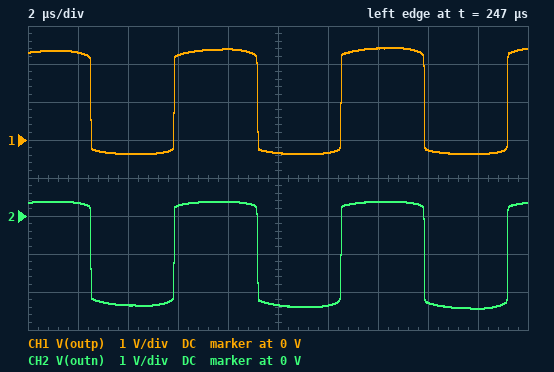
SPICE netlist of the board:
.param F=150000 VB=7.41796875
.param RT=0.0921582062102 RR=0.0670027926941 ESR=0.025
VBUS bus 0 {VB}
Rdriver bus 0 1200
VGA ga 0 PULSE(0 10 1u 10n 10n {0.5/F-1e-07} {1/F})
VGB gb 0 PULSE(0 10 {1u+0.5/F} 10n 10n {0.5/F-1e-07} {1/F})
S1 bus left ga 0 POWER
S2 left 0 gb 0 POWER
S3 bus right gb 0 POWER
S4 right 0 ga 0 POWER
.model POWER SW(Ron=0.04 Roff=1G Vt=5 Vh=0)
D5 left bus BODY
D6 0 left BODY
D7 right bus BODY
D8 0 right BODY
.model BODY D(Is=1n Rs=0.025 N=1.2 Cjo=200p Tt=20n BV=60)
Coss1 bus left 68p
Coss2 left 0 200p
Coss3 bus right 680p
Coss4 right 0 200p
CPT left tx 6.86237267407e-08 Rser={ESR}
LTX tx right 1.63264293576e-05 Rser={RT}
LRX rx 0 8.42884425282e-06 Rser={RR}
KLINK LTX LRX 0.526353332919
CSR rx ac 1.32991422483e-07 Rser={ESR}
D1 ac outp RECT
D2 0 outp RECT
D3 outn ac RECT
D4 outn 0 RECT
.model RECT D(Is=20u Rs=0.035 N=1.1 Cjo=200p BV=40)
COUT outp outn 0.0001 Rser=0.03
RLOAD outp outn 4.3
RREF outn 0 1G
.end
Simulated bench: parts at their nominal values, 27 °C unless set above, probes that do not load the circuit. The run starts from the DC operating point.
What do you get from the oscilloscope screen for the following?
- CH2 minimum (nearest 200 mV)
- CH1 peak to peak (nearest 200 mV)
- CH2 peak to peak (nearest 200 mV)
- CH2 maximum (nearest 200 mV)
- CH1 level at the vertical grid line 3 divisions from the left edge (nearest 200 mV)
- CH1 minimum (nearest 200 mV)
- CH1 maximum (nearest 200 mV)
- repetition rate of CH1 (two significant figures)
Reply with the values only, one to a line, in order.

-2.4 V
2.8 V
2.8 V
400 mV
2.2 V
-400 mV
2.4 V
150 kHz
